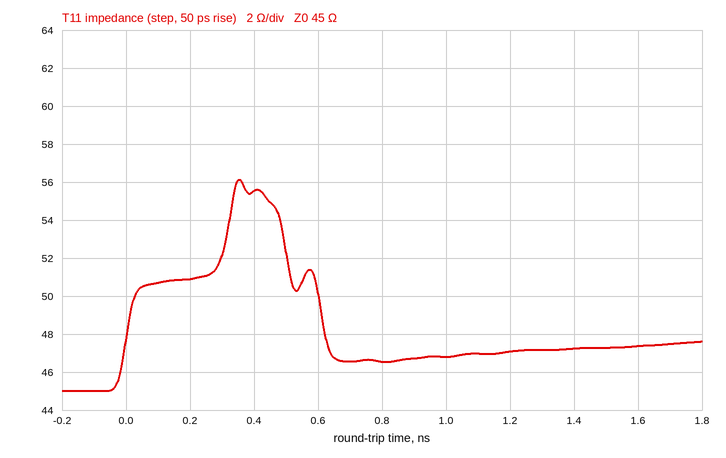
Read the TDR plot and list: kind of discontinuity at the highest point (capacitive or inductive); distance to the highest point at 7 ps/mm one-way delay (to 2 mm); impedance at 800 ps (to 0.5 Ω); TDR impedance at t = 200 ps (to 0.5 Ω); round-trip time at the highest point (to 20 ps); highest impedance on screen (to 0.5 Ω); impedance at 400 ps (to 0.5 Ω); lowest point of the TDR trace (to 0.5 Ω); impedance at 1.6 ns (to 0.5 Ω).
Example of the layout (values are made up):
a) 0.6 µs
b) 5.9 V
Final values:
a) inductive
b) 26 mm
c) 46.5 Ω
d) 51.0 Ω
e) 360 ps
f) 56.0 Ω
g) 55.5 Ω
h) 45.0 Ω
i) 47.5 Ω
